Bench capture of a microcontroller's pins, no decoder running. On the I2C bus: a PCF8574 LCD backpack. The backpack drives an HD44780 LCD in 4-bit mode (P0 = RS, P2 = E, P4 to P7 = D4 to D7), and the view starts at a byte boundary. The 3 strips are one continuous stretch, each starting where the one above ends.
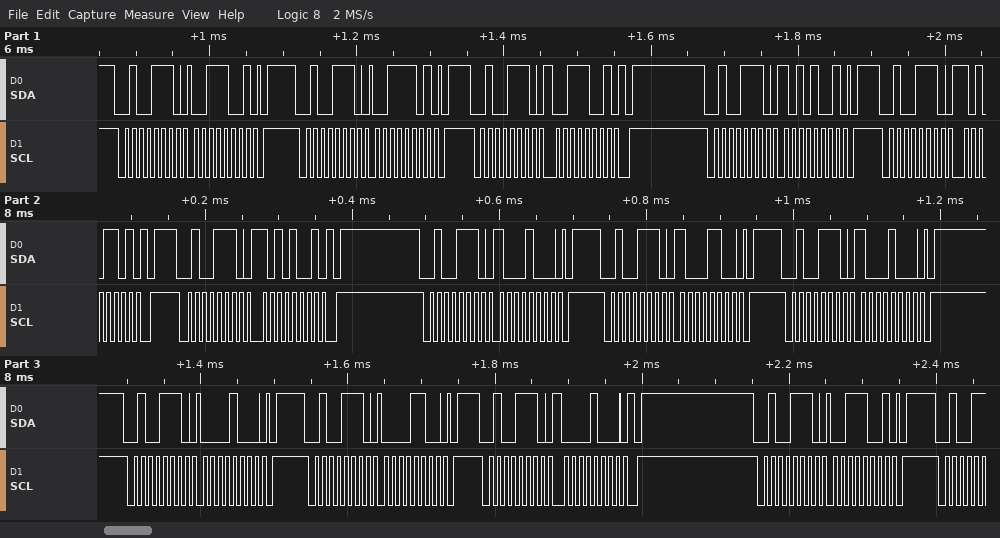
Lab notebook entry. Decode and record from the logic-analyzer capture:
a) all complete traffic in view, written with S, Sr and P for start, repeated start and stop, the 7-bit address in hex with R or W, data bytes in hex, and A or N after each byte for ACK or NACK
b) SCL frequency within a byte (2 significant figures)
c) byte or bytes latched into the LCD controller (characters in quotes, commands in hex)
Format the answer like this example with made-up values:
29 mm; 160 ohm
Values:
S 27W A 39 A P S 27W A 3D A P S 27W A 39 A P S 27W A A9 A P S 27W A AD A P S 27W A A9 A P S 27W A 88 A P S 27W A 8C A P S 27W A 88 A P S 27W A 08 A P S 27W A 0C A P S 27W A 08 A P S 27W A 39 A P; 100 kHz; ':' 0x80
